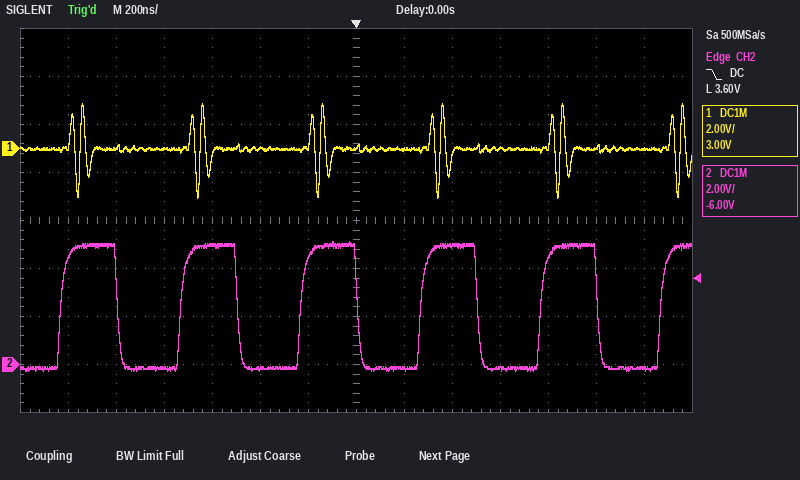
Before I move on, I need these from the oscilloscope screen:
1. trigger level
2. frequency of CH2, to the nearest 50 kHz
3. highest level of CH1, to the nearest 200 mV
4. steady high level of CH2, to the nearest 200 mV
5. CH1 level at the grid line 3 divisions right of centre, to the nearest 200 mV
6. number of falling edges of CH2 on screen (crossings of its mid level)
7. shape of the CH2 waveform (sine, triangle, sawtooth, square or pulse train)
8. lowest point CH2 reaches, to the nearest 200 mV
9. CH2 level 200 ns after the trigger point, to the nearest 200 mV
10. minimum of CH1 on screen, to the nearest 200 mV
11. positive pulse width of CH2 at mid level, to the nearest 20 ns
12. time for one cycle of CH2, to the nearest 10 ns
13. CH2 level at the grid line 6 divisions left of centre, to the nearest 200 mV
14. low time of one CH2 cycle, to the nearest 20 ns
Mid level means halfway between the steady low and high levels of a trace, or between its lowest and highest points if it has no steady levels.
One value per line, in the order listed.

3.60 V
2.00 MHz
1.8 V
5.0 V
0.0 V
5
square
-200 mV
-200 mV
-2.0 V
240 ns
500 ns
4.4 V
260 ns
